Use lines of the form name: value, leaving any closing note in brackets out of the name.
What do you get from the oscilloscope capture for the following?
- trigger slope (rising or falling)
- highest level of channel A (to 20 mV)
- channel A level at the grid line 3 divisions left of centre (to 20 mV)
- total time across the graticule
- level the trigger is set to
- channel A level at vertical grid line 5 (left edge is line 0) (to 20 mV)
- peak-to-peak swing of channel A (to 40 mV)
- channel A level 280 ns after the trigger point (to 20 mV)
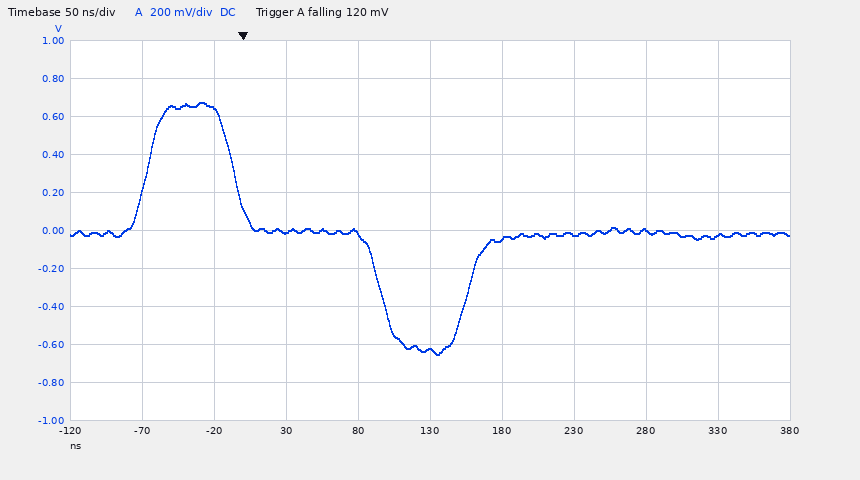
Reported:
trigger slope: falling
highest level of channel A: 680 mV
channel A level at the grid line 3 divisions left of centre: 640 mV
total time across the graticule: 500 ns
level the trigger is set to: 120 mV
channel A level at vertical grid line 5 (left edge is line 0): -620 mV
peak-to-peak swing of channel A: 1.32 V
channel A level 280 ns after the trigger point: 0 mV
